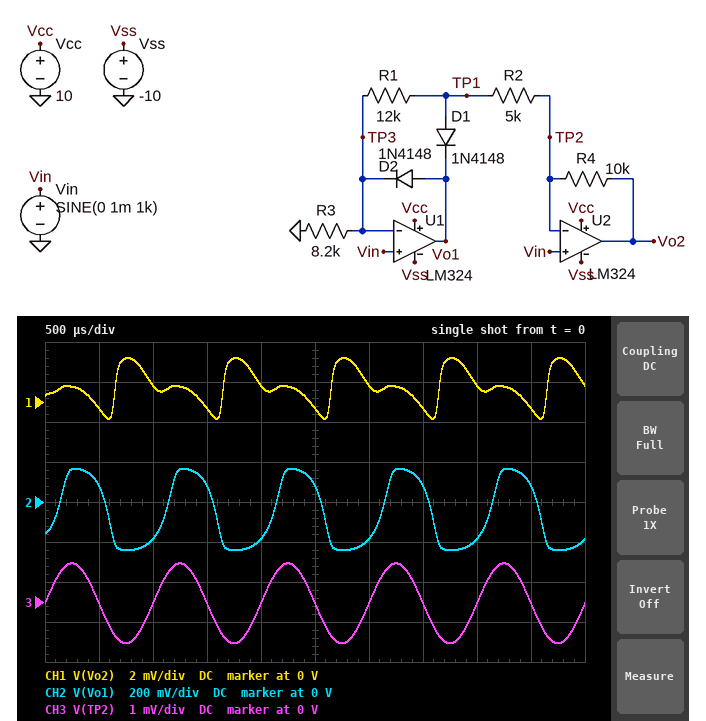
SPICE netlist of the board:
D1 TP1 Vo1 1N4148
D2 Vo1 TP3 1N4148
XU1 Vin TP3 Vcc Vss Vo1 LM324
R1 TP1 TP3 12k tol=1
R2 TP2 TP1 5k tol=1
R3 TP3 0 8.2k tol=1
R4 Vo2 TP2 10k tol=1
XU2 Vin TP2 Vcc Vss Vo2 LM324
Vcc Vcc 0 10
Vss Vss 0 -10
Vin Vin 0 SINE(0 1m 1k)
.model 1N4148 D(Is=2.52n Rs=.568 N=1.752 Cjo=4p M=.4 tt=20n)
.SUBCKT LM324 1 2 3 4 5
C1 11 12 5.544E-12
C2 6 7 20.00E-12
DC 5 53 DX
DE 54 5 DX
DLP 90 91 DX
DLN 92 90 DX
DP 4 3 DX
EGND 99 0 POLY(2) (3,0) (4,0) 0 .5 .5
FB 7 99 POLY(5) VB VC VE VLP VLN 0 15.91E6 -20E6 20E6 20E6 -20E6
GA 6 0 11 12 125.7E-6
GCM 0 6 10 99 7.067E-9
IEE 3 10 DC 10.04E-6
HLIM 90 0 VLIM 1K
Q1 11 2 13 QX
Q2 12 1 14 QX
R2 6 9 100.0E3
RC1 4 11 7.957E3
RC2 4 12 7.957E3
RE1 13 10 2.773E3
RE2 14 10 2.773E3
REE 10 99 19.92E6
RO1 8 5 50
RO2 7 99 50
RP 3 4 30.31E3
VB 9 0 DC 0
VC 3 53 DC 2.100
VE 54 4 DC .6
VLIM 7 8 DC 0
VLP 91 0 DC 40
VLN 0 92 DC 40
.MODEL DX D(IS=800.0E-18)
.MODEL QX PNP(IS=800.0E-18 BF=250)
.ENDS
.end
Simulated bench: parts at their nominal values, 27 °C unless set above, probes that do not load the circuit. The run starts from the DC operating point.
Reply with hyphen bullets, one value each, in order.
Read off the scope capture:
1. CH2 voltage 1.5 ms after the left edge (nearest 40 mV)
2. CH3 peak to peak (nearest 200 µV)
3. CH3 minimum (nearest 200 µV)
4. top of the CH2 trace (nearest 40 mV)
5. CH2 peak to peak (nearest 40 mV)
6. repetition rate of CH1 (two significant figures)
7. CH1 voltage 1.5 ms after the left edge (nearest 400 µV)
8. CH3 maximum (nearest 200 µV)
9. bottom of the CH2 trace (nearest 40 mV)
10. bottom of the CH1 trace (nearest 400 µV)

- 80 mV
- 2.0 mV
- -1.0 mV
- 160 mV
- 400 mV
- 1.0 kHz
- -400 µV
- 1.0 mV
- -240 mV
- -800 µV
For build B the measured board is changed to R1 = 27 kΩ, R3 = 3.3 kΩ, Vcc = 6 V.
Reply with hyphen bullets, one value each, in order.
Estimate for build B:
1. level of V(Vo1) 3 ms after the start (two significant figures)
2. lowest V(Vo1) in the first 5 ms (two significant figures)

- -260 mV
- -320 mV
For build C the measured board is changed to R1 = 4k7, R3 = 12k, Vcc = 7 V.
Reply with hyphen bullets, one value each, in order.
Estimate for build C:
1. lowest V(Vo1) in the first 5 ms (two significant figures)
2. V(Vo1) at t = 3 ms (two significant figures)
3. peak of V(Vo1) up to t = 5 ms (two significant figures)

- -200 mV
- -160 mV
- 130 mV
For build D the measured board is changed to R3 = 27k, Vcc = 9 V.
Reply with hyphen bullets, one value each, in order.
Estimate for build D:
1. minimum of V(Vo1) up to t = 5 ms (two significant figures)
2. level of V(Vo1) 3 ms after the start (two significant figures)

- -200 mV
- -160 mV
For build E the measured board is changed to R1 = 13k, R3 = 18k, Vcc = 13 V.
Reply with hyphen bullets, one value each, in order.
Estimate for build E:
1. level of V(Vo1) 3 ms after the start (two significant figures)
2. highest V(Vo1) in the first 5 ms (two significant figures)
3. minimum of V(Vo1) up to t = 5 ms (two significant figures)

- -160 mV
- 120 mV
- -210 mV
